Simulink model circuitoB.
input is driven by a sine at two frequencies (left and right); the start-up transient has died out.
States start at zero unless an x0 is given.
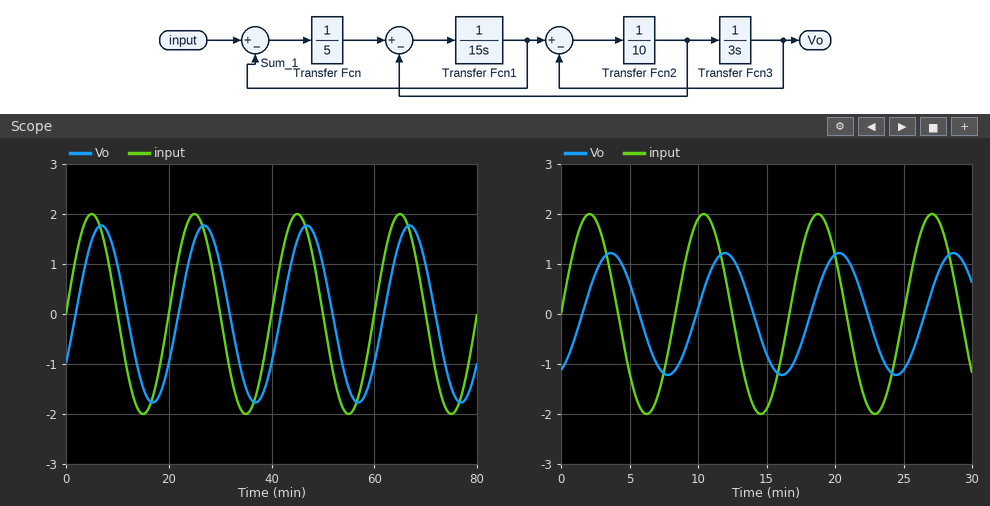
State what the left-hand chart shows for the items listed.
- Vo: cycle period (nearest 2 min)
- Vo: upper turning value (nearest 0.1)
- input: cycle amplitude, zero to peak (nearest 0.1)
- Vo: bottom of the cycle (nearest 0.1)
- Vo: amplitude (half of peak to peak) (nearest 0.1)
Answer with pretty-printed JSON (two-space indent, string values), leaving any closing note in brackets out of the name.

{
  "Vo: cycle period": "20 min",
  "Vo: upper turning value": "1.8",
  "input: cycle amplitude, zero to peak": "2.0",
  "Vo: bottom of the cycle": "-1.8",
  "Vo: amplitude (half of peak to peak)": "1.8"
}
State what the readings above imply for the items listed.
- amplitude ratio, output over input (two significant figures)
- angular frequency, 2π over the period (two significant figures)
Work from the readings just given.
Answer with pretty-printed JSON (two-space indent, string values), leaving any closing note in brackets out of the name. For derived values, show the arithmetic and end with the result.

{
  "amplitude ratio, output over input": "1.8 / 2 = 0.90",
  "angular frequency, 2π over the period": "2π / 20 = 0.31 rad/min"
}
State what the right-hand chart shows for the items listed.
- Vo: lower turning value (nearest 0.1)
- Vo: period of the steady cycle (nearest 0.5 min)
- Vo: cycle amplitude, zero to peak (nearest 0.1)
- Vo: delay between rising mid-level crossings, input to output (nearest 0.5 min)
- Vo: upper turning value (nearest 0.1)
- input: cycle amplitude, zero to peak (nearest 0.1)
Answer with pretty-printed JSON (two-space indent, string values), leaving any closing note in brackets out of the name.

{
  "Vo: lower turning value": "-1.2",
  "Vo: period of the steady cycle": "8.5 min",
  "Vo: cycle amplitude, zero to peak": "1.2",
  "Vo: delay between rising mid-level crossings, input to output": "1.5 min",
  "Vo: upper turning value": "1.2",
  "input: cycle amplitude, zero to peak": "2.0"
}
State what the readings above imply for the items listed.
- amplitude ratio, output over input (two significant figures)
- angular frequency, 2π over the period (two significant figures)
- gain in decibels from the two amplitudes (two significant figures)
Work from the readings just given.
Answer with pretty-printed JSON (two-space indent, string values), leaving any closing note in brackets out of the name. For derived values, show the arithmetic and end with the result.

{
  "amplitude ratio, output over input": "1.2 / 2 = 0.60",
  "angular frequency, 2π over the period": "2π / 8.5 = 0.74 rad/min",
  "gain in decibels from the two amplitudes": "20 log10(1.2 / 2) = -4.4 dB"
}
